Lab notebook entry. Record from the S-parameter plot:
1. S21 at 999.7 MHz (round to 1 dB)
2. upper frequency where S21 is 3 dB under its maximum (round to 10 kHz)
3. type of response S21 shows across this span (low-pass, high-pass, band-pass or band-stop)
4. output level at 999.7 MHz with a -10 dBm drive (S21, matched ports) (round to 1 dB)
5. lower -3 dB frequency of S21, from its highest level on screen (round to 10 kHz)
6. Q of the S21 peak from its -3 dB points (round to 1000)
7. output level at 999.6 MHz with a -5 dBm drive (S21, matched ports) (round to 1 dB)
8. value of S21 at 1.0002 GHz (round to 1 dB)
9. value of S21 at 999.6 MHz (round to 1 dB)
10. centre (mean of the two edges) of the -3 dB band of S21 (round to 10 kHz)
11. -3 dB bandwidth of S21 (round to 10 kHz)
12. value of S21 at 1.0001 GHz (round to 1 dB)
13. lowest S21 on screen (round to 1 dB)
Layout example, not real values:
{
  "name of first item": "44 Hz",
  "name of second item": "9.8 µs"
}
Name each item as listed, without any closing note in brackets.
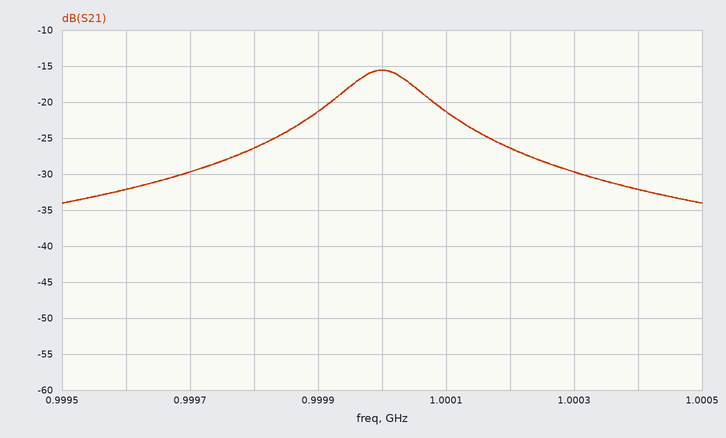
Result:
{
  "S21 at 999.7 MHz": "-30 dB",
  "upper frequency where S21 is 3 dB under its maximum": "1.00006 GHz",
  "type of response S21 shows across this span": "band-pass",
  "output level at 999.7 MHz with a -10 dBm drive (S21, matched ports)": "-40 dBm",
  "lower -3 dB frequency of S21, from its highest level on screen": "999.94 MHz",
  "Q of the S21 peak from its -3 dB points": "8000",
  "output level at 999.6 MHz with a -5 dBm drive (S21, matched ports)": "-37 dBm",
  "value of S21 at 1.0002 GHz": "-26 dB",
  "value of S21 at 999.6 MHz": "-32 dB",
  "centre (mean of the two edges) of the -3 dB band of S21": "1.00000 GHz",
  "-3 dB bandwidth of S21": "120 kHz",
  "value of S21 at 1.0001 GHz": "-21 dB",
  "lowest S21 on screen": "-34 dB"
}
